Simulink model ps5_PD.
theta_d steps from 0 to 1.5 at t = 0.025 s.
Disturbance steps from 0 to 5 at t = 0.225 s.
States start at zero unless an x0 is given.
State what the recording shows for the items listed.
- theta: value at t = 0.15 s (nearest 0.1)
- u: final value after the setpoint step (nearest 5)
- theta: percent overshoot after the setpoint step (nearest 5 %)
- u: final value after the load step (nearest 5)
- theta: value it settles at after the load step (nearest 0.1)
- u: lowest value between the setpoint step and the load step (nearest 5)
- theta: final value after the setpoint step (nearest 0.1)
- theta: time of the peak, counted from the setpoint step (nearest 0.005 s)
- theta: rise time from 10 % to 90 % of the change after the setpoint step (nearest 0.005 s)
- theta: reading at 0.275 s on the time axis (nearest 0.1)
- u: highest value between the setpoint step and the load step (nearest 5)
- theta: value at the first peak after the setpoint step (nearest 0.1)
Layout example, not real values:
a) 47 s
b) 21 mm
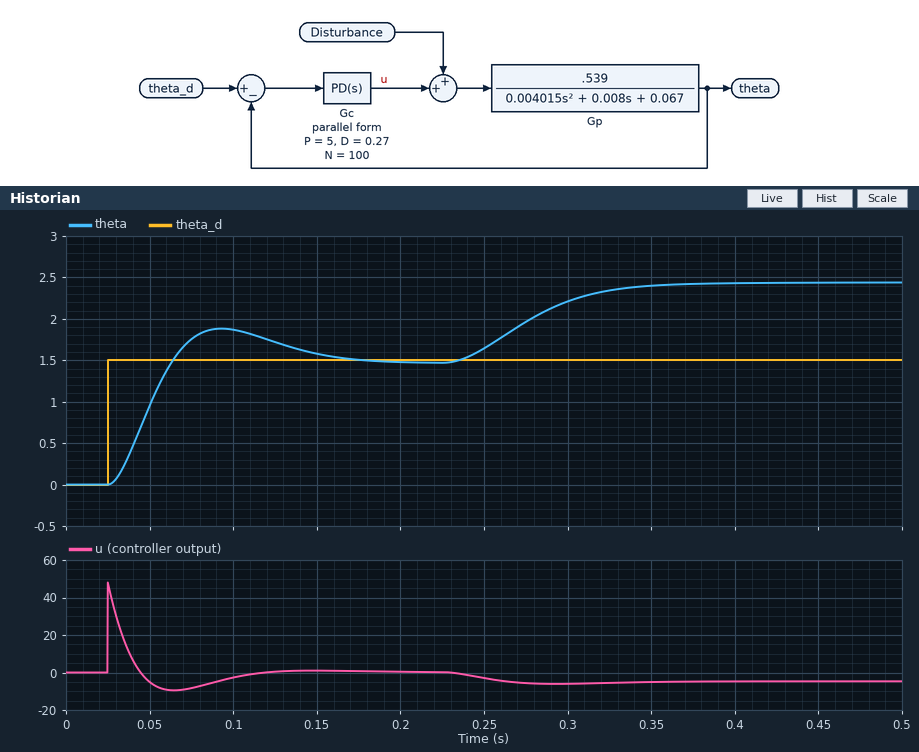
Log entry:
a) 1.6
b) 0
c) 30 %
d) -5
e) 2.4
f) -10
g) 1.5
h) 0.070 s
i) 0.025 s
j) 2.0
k) 50
l) 1.9
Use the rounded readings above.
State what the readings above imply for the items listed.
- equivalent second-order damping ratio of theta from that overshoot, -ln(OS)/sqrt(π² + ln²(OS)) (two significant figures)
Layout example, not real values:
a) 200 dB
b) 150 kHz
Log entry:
a) 0.36
